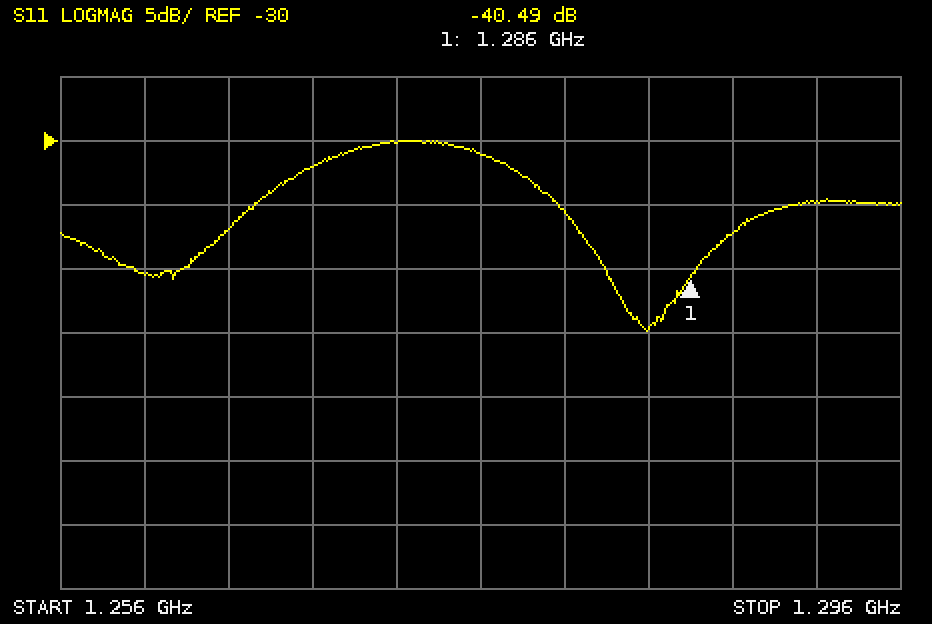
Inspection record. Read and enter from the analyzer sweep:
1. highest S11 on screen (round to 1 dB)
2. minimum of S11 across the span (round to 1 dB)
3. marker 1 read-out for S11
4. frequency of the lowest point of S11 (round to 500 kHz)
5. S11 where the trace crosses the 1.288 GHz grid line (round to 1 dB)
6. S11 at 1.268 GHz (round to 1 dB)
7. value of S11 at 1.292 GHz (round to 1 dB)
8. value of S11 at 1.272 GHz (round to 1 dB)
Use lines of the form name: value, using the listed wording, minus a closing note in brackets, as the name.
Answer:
highest S11 on screen: -30 dB
minimum of S11 across the span: -45 dB
marker 1 read-out for S11: -40.49 dB
frequency of the lowest point of S11: 1.2840 GHz
S11 where the trace crosses the 1.288 GHz grid line: -37 dB
S11 at 1.268 GHz: -32 dB
value of S11 at 1.292 GHz: -35 dB
value of S11 at 1.272 GHz: -30 dB
